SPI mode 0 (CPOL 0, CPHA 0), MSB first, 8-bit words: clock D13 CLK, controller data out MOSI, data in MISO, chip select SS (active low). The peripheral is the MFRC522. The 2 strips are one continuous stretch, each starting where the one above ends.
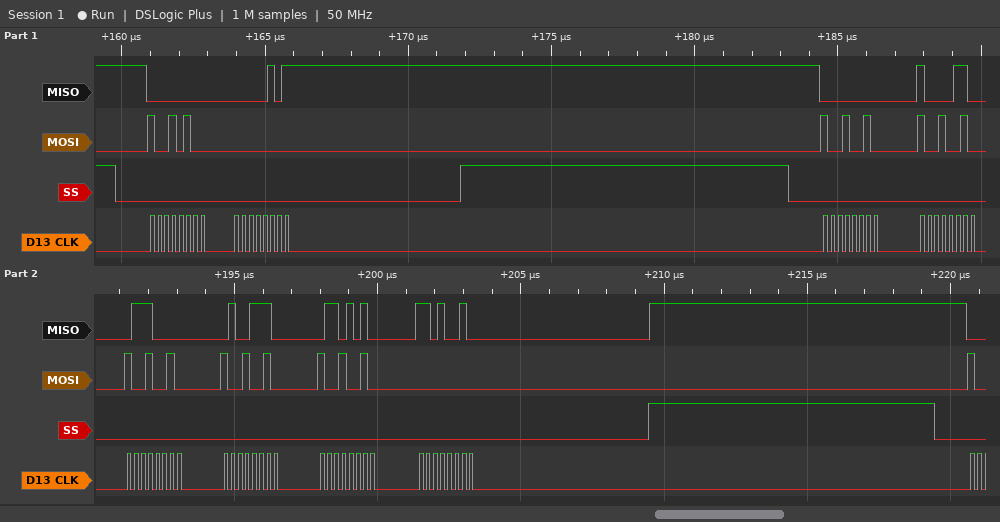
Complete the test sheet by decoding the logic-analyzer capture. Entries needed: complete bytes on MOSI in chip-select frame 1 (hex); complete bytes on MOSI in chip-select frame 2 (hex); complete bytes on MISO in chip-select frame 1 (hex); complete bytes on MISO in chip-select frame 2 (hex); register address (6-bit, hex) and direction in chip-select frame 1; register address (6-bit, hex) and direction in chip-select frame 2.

94 00
92 92 92 92 92 00
00 05
00 86 70 4E 6A D2
0x0A read
0x09 read
